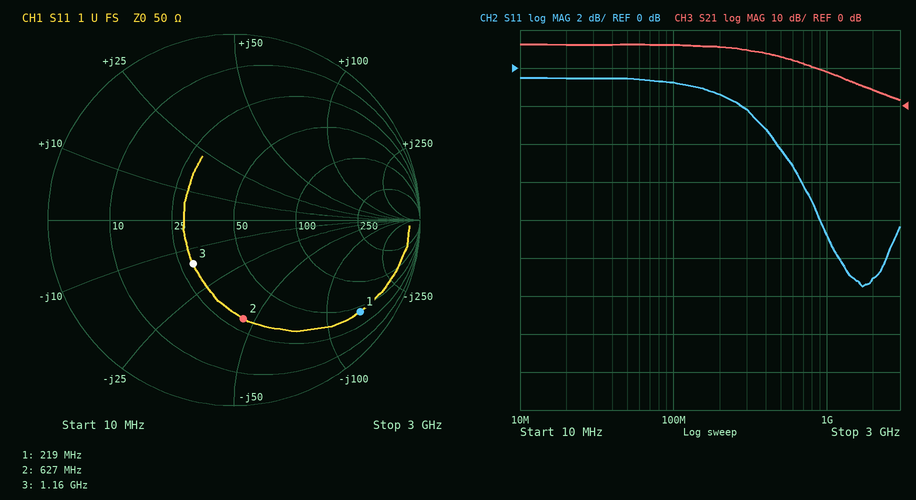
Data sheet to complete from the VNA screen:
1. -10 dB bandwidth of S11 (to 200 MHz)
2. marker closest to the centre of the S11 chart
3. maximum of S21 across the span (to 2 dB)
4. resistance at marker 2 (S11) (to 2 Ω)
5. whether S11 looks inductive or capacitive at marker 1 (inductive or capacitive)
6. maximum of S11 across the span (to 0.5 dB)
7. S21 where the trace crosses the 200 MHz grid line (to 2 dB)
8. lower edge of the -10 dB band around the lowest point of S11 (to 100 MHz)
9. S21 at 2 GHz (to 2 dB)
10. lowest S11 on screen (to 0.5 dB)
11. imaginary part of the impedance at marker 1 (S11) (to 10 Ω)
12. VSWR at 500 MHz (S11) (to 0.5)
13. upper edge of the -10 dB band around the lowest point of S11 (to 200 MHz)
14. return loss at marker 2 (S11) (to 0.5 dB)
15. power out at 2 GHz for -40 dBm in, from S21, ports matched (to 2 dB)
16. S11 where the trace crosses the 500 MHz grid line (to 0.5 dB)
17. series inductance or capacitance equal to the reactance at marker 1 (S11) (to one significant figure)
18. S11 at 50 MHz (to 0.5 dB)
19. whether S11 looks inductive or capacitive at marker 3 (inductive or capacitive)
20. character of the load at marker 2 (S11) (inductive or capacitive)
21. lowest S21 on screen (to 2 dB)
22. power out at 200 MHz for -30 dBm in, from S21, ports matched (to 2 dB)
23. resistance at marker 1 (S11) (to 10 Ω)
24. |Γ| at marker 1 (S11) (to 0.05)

1.2 GHz
marker 3
16 dB
30 Ω
capacitive
-0.5 dB
16 dB
1.2 GHz
4 dB
-11.5 dB
-140 Ω
4.0
2.4 GHz
5.5 dB
-36 dBm
-4.5 dB
5 pF
-0.5 dB
capacitive
capacitive
2 dB
-14 dBm
40 Ω
0.85
